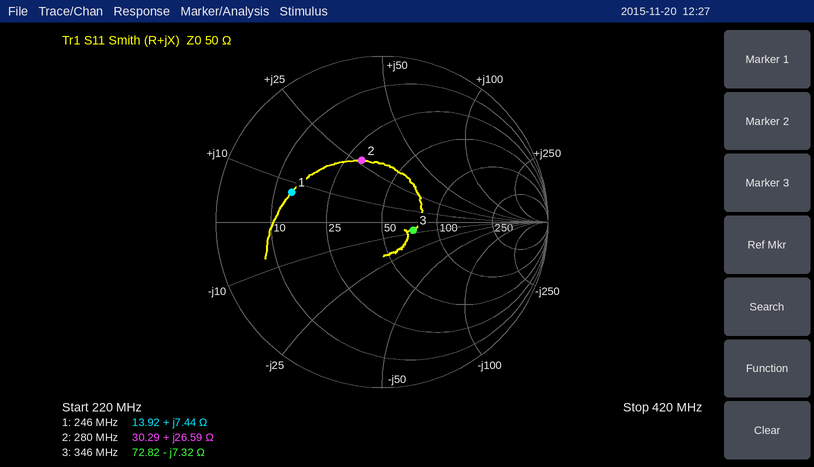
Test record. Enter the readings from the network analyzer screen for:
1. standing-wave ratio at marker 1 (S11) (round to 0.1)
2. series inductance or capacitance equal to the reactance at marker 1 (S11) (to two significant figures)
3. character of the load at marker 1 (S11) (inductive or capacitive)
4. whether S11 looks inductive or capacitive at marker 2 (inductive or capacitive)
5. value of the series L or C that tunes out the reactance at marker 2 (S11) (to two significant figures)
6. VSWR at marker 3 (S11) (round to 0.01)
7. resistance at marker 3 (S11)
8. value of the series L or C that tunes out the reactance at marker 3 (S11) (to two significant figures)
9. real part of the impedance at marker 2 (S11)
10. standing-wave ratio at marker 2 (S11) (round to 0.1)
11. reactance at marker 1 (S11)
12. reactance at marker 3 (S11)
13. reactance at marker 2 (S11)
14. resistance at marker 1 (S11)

3.7
4.8 nH
inductive
inductive
21 pF
1.48
72.82 Ω
3.4 nH
30.29 Ω
2.3
+7.44 Ω
-7.32 Ω
+26.59 Ω
13.92 Ω
